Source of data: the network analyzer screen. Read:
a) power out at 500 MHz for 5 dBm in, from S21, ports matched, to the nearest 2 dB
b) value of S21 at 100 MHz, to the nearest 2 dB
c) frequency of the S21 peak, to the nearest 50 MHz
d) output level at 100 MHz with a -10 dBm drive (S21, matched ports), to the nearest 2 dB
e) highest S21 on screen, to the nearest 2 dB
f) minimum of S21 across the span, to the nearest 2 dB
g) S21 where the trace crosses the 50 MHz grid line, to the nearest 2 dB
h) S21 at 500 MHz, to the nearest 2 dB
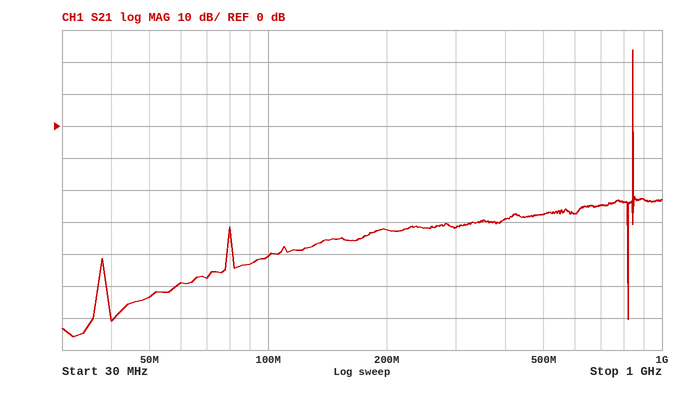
-22 dBm
-40 dB
850 MHz
-50 dBm
24 dB
-66 dB
-54 dB
-28 dB
